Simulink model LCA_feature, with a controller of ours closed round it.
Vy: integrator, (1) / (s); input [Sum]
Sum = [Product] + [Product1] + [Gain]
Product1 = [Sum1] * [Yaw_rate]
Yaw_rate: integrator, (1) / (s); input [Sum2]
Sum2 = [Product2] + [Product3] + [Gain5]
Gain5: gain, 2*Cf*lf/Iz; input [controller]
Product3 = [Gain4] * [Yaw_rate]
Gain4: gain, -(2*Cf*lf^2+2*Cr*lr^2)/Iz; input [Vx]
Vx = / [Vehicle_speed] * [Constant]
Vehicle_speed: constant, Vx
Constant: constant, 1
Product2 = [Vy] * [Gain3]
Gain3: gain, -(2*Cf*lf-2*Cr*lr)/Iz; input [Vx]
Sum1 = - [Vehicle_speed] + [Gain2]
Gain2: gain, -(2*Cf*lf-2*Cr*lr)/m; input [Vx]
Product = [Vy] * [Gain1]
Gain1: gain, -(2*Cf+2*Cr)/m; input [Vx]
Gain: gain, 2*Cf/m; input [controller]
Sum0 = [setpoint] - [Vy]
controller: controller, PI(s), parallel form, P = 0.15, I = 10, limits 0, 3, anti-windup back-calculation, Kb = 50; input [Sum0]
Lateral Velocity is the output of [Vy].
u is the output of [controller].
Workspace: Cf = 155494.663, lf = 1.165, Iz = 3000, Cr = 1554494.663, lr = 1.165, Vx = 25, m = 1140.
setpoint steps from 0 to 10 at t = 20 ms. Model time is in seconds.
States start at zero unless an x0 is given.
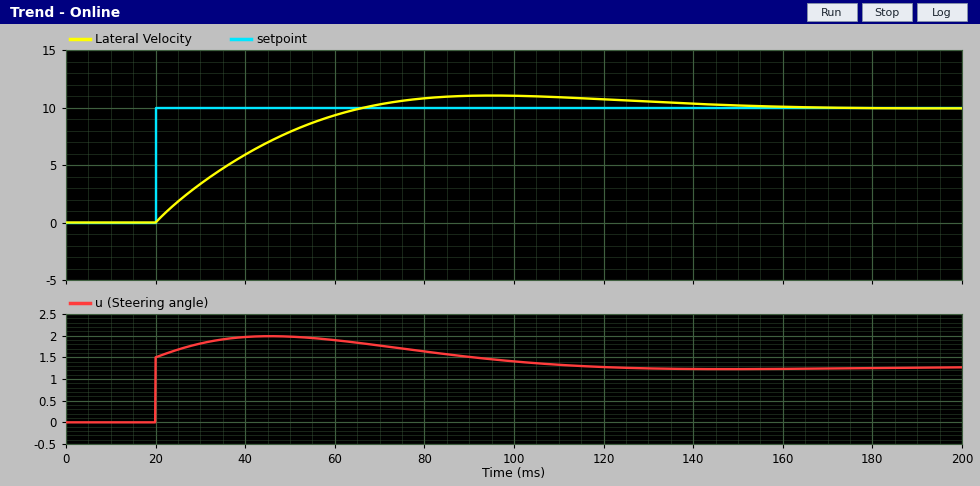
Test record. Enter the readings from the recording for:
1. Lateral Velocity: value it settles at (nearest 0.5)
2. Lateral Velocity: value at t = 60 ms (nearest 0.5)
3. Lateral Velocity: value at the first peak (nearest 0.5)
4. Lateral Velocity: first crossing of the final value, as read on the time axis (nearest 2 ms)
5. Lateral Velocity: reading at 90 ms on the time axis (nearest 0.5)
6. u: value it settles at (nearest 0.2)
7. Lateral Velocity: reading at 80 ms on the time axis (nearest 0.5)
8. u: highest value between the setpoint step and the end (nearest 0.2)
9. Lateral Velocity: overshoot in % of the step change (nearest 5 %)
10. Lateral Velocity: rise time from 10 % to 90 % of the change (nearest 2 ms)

10.0
9.5
11.0
66 ms
11.0
1.2
11.0
2.0
10 %
34 ms
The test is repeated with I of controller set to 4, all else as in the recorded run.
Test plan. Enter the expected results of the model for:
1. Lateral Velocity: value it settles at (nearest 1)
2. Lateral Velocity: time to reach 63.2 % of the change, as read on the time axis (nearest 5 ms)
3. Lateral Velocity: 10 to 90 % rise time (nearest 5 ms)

10
55 ms
75 ms
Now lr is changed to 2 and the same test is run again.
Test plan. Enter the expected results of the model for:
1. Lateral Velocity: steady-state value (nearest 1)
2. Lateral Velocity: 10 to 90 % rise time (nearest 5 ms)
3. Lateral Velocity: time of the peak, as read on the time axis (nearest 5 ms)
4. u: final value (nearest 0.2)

10
25 ms
80 ms
1.0
